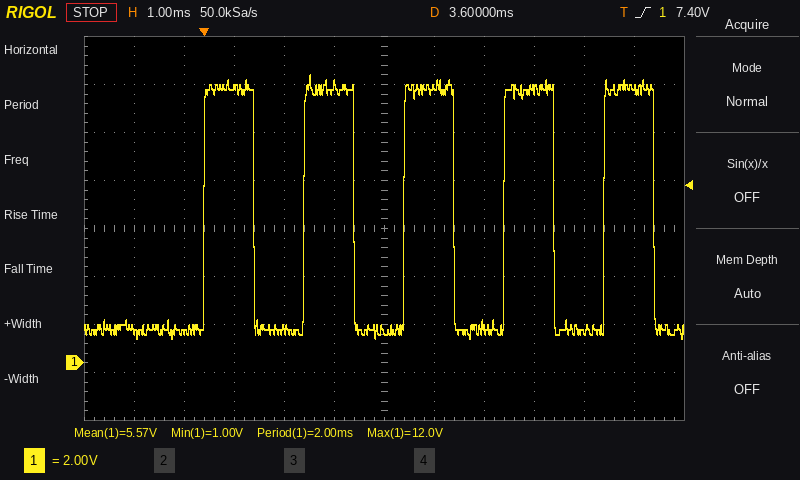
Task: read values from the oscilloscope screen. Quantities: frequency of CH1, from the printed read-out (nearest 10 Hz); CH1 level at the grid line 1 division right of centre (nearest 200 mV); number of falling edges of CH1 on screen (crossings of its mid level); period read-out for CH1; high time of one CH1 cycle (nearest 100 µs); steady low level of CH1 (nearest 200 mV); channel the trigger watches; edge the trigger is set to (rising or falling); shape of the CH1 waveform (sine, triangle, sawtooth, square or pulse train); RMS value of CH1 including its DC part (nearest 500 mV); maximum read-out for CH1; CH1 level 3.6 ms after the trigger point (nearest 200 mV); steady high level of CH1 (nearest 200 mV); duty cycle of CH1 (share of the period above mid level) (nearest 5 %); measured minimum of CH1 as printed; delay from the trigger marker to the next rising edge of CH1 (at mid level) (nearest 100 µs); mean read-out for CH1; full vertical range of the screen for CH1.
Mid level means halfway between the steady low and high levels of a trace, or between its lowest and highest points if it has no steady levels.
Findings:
500 Hz
11.6 V
5
2.00 ms
1.0 ms
1.4 V
CH1
rising
square
8.0 V
12.0 V
1.4 V
11.4 V
50 %
1.00 V
2.0 ms
5.57 V
16 V
